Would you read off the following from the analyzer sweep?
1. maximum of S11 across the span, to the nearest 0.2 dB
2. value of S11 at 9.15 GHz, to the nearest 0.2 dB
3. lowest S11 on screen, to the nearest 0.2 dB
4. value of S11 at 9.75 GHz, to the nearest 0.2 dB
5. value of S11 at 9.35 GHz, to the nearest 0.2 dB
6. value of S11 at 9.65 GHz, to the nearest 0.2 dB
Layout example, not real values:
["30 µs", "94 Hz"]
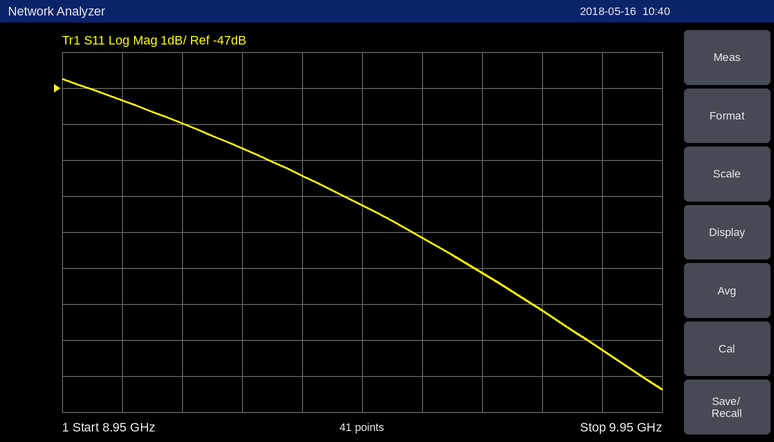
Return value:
["-46.8 dB", "-48.0 dB", "-55.4 dB", "-53.2 dB", "-49.4 dB", "-52.2 dB"]
